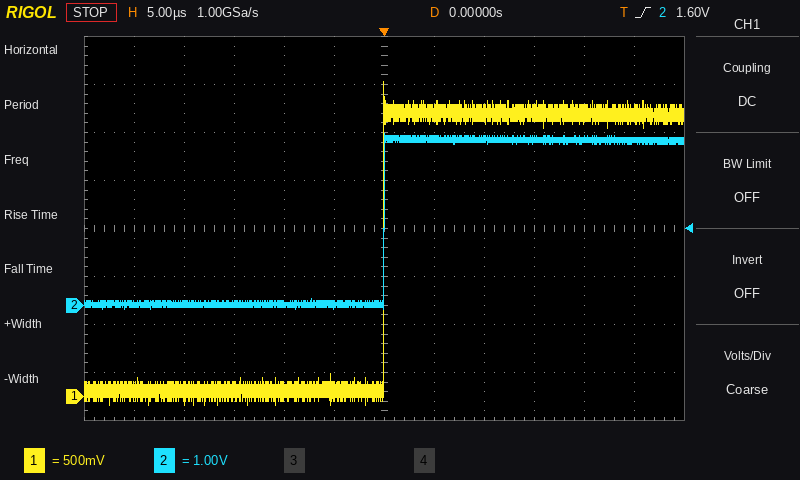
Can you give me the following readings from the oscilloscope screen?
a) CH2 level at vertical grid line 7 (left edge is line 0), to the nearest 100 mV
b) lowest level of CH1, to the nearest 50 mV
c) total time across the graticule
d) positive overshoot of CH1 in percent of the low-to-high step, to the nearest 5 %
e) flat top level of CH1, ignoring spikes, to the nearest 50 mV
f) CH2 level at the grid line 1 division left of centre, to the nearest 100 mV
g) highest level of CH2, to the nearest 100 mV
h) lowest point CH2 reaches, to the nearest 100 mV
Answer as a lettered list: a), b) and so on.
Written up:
a) 3.5 V
b) -100 mV
c) 60 µs
d) 10 %
e) 2.95 V
f) 0.0 V
g) 3.6 V
h) -100 mV
